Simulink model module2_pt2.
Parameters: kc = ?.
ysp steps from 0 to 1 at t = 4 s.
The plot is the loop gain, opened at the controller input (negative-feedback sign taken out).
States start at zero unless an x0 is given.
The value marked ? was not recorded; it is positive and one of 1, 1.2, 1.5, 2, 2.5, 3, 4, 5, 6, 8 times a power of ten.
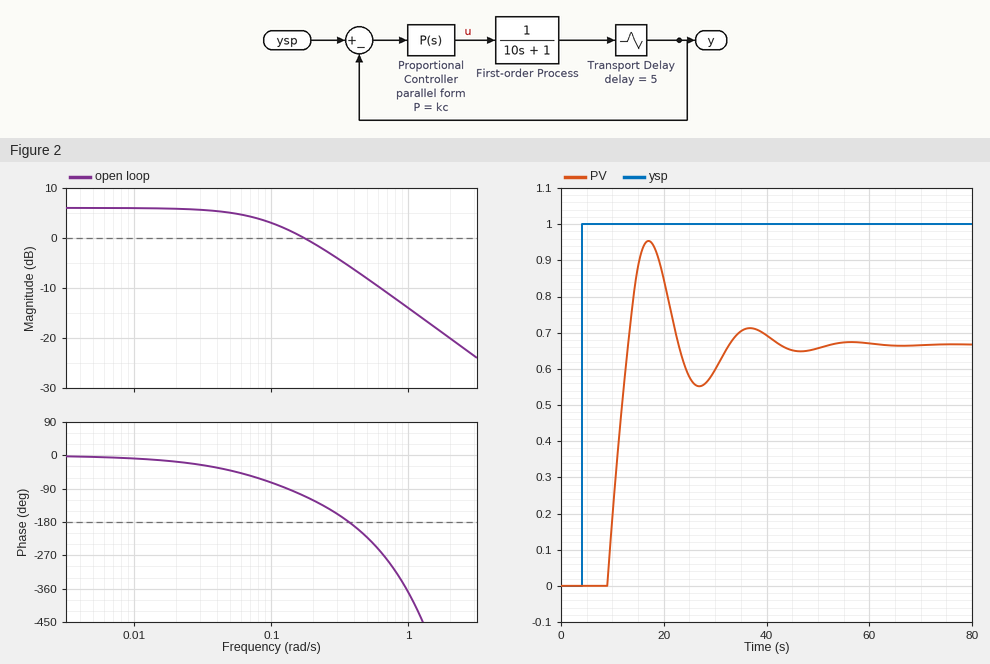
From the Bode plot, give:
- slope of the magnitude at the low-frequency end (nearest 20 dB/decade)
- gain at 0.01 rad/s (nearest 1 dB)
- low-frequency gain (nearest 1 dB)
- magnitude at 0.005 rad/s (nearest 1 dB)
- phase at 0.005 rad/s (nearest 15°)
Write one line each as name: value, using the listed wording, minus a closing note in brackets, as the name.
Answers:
slope of the magnitude at the low-frequency end: 0 dB/decade
gain at 0.01 rad/s: 6 dB
low-frequency gain: 6 dB
magnitude at 0.005 rad/s: 6 dB
phase at 0.005 rad/s: 0°
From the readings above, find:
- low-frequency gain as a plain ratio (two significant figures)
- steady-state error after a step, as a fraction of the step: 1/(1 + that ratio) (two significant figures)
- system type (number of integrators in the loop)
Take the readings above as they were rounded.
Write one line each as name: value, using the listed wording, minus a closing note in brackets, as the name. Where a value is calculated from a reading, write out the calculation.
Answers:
low-frequency gain as a plain ratio: 10^(6 / 20) = 2.0
steady-state error after a step, as a fraction of the step: 1/(1 + that ratio): 1 / (1 + 2) = 0.33
system type: 0
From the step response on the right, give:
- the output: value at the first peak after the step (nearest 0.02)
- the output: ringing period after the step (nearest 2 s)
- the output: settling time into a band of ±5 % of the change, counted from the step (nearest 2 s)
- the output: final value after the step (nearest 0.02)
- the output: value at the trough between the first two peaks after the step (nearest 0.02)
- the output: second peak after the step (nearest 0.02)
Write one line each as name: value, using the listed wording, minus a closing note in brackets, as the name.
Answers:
the output: value at the first peak after the step: 0.96
the output: ringing period after the step: 20 s
the output: settling time into a band of ±5 % of the change, counted from the step: 36 s
the output: final value after the step: 0.66
the output: value at the trough between the first two peaks after the step: 0.56
the output: second peak after the step: 0.72
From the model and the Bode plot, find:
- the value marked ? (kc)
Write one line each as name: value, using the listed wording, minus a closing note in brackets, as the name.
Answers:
the value marked ?: 2
